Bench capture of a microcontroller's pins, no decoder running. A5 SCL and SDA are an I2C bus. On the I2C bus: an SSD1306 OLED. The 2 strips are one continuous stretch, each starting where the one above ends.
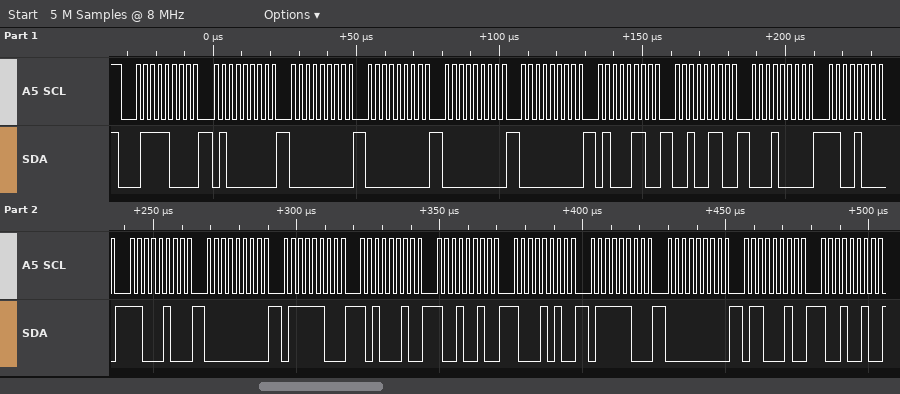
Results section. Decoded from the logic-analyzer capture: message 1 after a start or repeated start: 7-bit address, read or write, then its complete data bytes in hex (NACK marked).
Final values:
0x3C write: 40 00 00 00 00 46 26 10 C8 C4 00 7C A2 92 8A 7C 00 62 92
